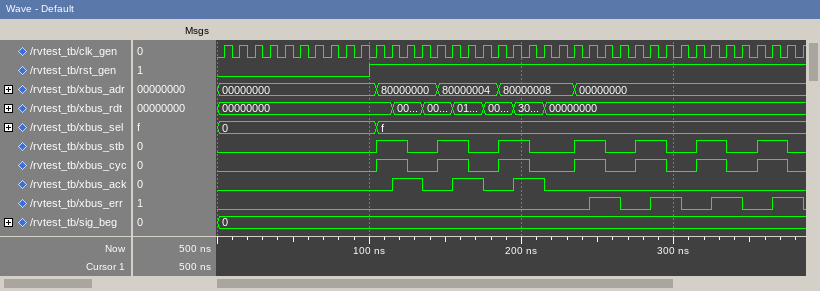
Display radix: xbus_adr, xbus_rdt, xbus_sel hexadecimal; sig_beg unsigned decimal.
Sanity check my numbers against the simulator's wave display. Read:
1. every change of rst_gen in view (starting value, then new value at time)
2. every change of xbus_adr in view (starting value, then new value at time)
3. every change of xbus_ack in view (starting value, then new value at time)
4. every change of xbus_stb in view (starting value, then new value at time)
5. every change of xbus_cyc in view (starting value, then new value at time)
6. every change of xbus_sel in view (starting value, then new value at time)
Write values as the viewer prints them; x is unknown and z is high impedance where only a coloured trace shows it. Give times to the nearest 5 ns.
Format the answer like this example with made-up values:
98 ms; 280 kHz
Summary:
0, 1 at 100 ns; 00000000, 80000000 at 105 ns, 80000004 at 145 ns, 80000008 at 185 ns, 00000000 at 235 ns; 0, 1 at 115 ns, 0 at 135 ns, 1 at 155 ns, 0 at 175 ns, 1 at 195 ns, 0 at 215 ns; 0, 1 at 105 ns, 0 at 125 ns, 1 at 145 ns, 0 at 165 ns, 1 at 185 ns, 0 at 205 ns, 1 at 235 ns, 0 at 255 ns, 1 at 275 ns, 0 at 295 ns, 1 at 315 ns, 0 at 335 ns, 1 at 355 ns, 0 at 375 ns; 0, 1 at 105 ns, 0 at 125 ns, 1 at 145 ns, 0 at 165 ns, 1 at 185 ns, 0 at 205 ns, 1 at 235 ns, 0 at 255 ns, 1 at 275 ns, 0 at 295 ns, 1 at 315 ns, 0 at 335 ns, 1 at 355 ns, 0 at 375 ns; 0, f at 105 ns
